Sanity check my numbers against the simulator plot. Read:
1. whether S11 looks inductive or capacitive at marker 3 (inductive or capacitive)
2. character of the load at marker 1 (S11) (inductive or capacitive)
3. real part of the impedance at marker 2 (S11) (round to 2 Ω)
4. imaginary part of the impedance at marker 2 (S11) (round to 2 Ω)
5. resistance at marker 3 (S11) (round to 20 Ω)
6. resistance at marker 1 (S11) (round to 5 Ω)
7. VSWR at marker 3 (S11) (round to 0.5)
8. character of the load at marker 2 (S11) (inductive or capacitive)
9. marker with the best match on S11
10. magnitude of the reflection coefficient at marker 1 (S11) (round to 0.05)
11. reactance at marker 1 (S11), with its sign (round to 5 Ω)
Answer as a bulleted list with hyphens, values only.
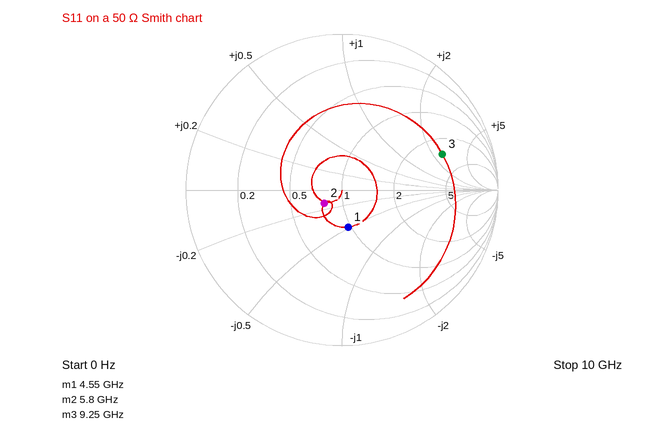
- inductive
- capacitive
- 40 Ω
- -6 Ω
- 140 Ω
- 50 Ω
- 5.5
- capacitive
- marker 2
- 0.25
- -25 Ω
